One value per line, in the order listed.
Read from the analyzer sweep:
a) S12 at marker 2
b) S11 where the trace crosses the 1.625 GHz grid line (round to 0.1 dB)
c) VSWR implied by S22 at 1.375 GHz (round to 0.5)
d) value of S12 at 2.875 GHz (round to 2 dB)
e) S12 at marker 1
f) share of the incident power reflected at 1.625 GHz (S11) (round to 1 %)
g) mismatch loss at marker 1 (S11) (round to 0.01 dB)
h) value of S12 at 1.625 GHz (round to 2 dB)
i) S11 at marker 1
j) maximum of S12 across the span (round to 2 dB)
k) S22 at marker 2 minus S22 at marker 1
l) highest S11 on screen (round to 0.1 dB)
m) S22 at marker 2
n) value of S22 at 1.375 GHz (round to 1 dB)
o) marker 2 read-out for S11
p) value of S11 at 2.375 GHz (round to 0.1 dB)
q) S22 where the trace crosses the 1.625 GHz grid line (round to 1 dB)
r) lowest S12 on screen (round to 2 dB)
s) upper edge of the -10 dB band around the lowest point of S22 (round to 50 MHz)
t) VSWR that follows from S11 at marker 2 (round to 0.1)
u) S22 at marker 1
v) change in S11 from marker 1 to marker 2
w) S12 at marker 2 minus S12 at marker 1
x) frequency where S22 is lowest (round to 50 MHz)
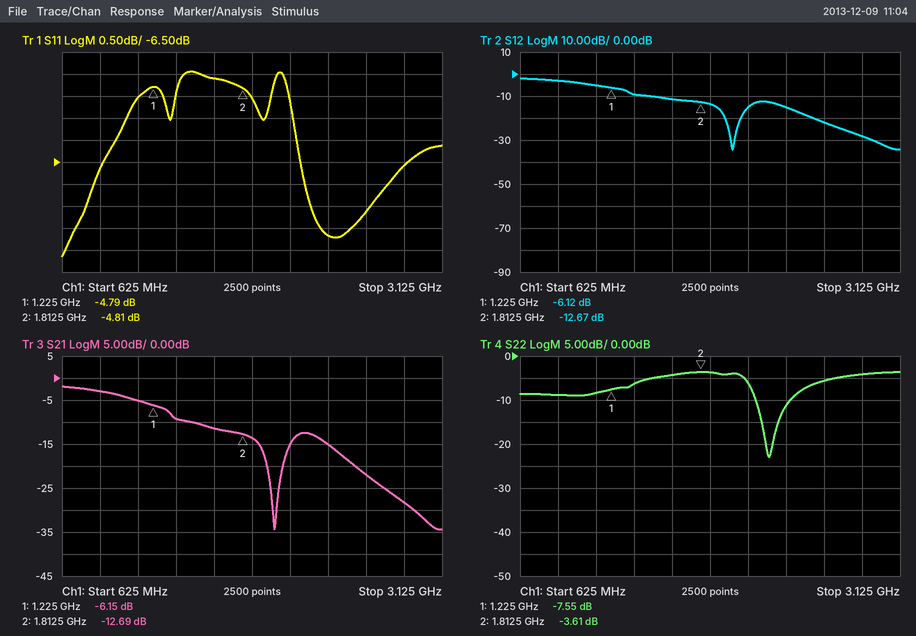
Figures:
-12.67 dB
-4.6 dB
3.0
-28 dB
-6.12 dB
35 %
1.75 dB
-12 dB
-4.79 dB
-2 dB
3.94 dB
-4.4 dB
-3.61 dB
-6 dB
-4.81 dB
-8.2 dB
-4 dB
-34 dB
2.40 GHz
3.7
-7.55 dB
-0.02 dB
-6.55 dB
2.25 GHz
